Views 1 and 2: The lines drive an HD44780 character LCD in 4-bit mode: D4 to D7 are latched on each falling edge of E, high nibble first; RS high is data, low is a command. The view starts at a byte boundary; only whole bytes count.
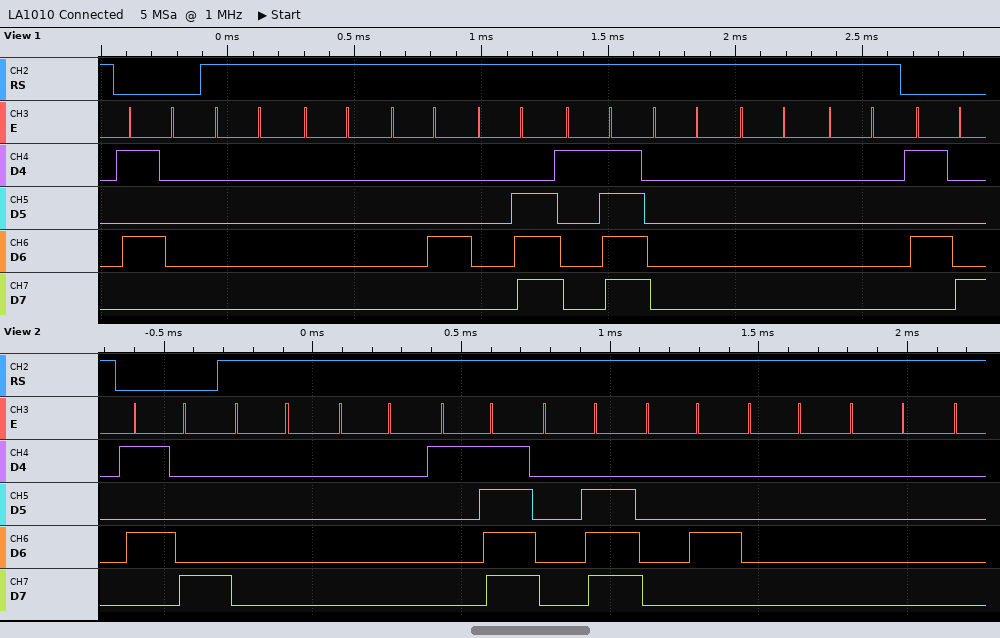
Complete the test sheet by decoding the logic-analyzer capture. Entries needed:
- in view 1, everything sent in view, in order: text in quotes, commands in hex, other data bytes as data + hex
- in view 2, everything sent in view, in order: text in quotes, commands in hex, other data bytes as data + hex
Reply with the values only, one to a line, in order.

0x50 data 00 00 04 0E 1F 00 00 00 0x58
0x58 data 00 00 1F 0E 04 00 00
